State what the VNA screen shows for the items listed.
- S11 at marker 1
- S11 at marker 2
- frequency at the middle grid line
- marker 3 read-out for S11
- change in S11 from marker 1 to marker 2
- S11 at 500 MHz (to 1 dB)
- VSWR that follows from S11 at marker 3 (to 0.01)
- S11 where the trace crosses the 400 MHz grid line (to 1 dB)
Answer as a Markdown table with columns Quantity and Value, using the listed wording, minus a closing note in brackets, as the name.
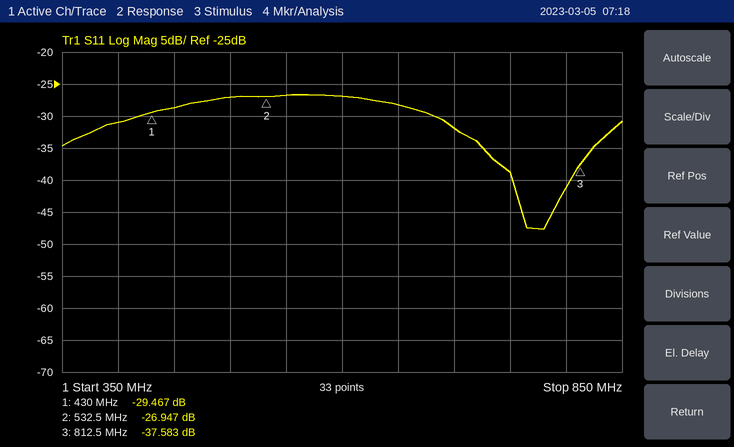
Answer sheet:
| Quantity | Value |
|---|---|
| S11 at marker 1 | -29.467 dB |
| S11 at marker 2 | -26.947 dB |
| frequency at the middle grid line | 600 MHz |
| marker 3 read-out for S11 | -37.583 dB |
| change in S11 from marker 1 to marker 2 | 2.520 dB |
| S11 at 500 MHz | -27 dB |
| VSWR that follows from S11 at marker 3 | 1.03 |
| S11 where the trace crosses the 400 MHz grid line | -31 dB |
